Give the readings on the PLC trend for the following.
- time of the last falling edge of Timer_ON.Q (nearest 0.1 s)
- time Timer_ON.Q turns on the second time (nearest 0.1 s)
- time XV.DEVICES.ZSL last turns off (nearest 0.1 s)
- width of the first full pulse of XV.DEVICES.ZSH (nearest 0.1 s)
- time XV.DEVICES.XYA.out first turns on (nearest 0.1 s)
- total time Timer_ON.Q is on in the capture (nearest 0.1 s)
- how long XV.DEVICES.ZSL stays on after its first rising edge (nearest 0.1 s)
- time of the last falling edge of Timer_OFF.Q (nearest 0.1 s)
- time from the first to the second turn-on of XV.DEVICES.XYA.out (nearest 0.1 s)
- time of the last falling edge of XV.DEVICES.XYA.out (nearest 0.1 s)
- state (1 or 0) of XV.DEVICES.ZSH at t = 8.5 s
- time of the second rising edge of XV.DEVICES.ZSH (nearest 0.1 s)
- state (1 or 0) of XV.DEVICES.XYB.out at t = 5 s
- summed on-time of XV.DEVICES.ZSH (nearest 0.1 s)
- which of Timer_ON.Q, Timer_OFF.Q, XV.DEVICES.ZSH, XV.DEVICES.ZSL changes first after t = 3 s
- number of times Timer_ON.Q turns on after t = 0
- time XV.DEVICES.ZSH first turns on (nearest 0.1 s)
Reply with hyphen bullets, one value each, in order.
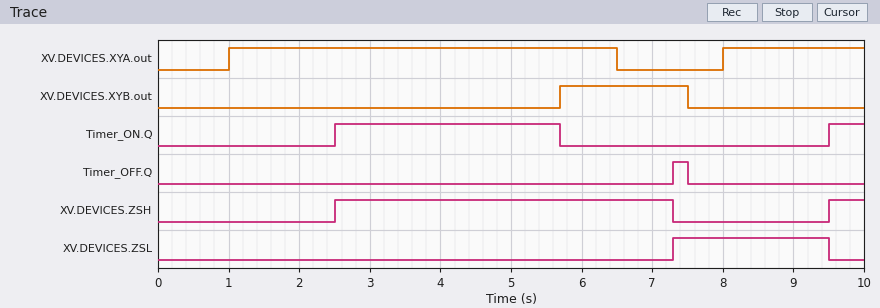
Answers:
- 5.7 s
- 9.5 s
- 9.5 s
- 4.8 s
- 1.0 s
- 3.7 s
- 2.2 s
- 7.5 s
- 7.0 s
- 6.5 s
- 0
- 9.5 s
- 0
- 5.3 s
- Timer_ON.Q
- 2
- 2.5 s
